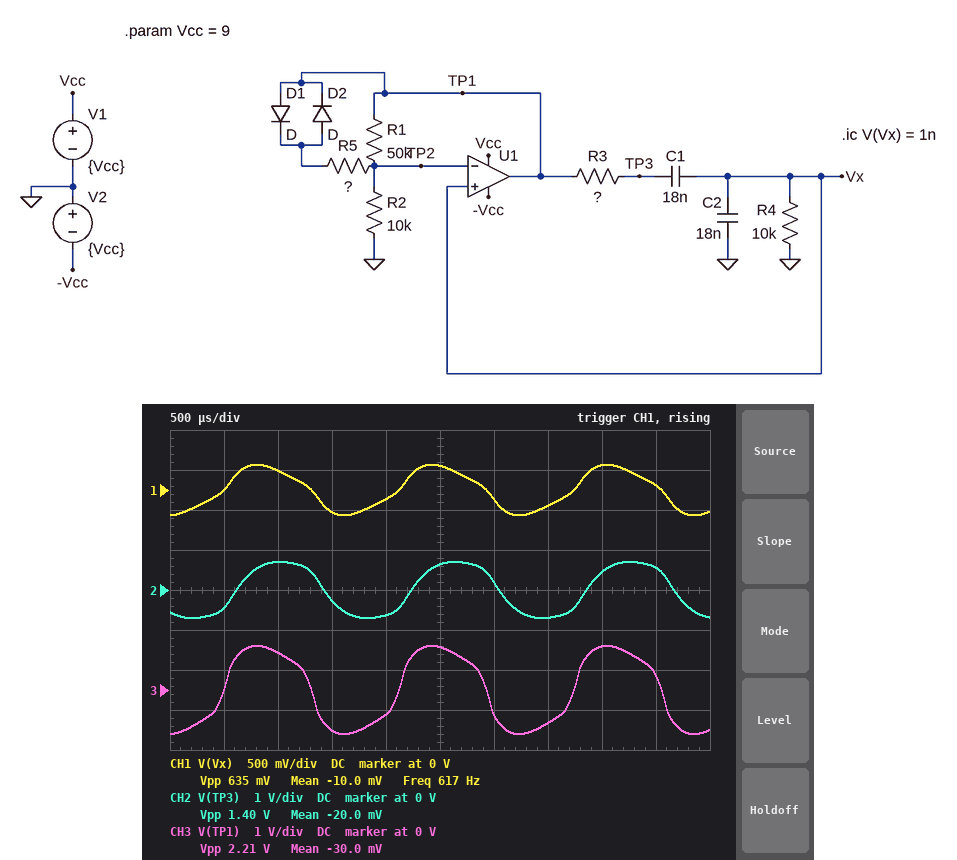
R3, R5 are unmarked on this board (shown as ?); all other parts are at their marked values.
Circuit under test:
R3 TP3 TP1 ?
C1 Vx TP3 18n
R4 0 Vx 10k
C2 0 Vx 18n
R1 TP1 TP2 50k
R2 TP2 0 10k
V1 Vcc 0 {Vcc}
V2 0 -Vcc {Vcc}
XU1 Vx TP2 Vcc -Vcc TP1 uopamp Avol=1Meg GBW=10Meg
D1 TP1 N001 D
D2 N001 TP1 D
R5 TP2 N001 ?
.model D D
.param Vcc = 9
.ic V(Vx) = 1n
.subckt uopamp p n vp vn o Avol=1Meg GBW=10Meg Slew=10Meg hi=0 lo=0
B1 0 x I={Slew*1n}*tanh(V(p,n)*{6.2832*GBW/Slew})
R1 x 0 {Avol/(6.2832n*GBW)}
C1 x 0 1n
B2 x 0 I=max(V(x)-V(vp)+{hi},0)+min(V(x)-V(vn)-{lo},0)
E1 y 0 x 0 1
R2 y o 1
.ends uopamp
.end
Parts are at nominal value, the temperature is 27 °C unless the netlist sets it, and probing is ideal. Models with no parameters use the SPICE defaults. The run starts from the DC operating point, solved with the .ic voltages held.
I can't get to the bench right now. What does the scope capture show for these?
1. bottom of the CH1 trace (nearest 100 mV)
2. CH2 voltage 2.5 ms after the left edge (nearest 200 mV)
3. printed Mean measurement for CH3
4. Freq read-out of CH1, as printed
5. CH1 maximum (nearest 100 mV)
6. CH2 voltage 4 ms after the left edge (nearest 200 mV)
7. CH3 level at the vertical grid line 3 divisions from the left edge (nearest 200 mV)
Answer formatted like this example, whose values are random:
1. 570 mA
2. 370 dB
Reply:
1. -300 mV
2. 600 mV
3. -30.0 mV
4. 617 Hz
5. 300 mV
6. 400 mV
7. -1.0 V
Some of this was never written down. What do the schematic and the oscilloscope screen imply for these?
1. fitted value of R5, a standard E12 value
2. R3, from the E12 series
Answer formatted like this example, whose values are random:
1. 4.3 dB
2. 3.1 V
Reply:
1. 15 kΩ
2. 18 kΩ
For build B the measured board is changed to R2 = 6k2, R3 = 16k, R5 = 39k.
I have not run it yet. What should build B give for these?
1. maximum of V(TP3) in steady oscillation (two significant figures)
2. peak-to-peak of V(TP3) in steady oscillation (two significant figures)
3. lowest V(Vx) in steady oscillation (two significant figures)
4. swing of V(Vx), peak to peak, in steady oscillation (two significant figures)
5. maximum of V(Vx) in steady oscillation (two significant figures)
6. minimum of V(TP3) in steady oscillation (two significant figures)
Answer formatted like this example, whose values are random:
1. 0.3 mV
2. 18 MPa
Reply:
1. 7.0 V
2. 14 V
3. -3.0 V
4. 6.0 V
5. 3.0 V
6. -7.0 V
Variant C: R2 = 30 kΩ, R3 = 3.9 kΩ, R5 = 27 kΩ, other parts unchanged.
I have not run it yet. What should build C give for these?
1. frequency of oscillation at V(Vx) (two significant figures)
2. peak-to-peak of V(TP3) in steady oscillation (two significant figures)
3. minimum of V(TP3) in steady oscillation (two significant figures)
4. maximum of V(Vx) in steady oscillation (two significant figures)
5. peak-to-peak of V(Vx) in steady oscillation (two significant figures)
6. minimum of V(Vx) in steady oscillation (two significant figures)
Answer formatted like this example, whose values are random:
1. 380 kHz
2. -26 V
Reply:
1. 1.4 kHz
2. 1.9 V
3. -950 mV
4. 480 mV
5. 950 mV
6. -480 mV
